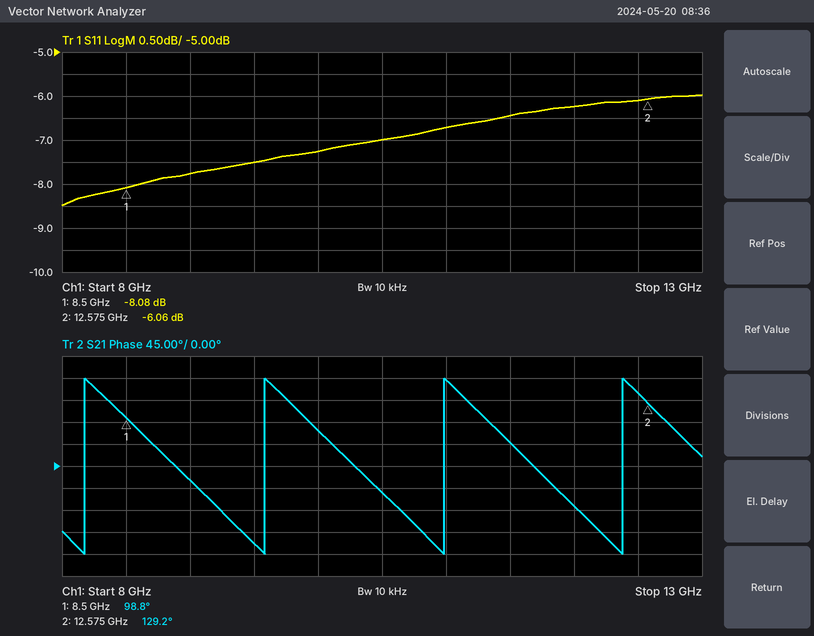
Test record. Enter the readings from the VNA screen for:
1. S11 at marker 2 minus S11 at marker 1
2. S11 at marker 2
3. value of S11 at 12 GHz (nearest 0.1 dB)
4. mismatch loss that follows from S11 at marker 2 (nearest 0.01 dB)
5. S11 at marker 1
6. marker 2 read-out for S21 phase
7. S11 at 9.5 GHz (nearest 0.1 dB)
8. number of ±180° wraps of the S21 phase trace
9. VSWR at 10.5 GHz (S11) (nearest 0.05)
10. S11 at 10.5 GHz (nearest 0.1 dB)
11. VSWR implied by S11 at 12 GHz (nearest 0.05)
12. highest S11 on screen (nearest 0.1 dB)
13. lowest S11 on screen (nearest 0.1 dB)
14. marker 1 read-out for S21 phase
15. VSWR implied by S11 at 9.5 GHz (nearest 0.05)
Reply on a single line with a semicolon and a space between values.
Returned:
2.02 dB; -6.06 dB; -6.2 dB; 1.24 dB; -8.08 dB; 129.2°; -7.5 dB; 4; 2.60; -7.0 dB; 2.90; -6.0 dB; -8.5 dB; 98.8°; 2.45
